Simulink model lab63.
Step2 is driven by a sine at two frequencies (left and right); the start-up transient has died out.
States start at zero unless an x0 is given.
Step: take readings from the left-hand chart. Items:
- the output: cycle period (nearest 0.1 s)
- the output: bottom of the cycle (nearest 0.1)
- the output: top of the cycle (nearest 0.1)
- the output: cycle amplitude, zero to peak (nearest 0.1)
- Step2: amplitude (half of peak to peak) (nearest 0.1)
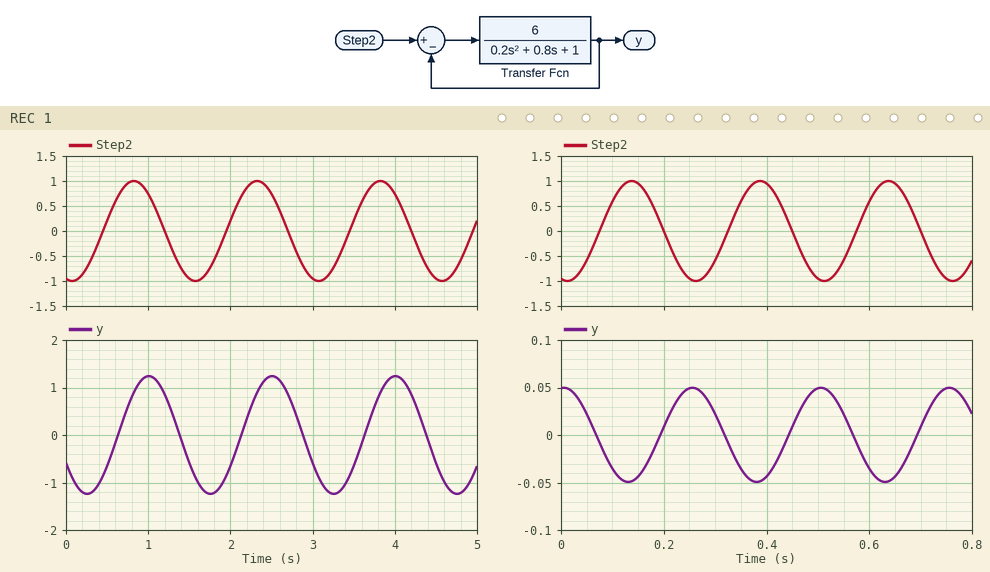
1.5 s
-1.2
1.2
1.2
1.0
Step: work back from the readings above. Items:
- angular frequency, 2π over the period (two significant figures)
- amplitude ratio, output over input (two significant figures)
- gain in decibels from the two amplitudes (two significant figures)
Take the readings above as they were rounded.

4.2 rad/s
1.2
1.6 dB
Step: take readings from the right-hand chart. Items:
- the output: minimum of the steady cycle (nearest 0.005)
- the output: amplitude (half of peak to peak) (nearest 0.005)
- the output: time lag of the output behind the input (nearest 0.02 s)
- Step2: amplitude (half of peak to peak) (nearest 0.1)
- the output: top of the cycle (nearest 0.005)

-0.050
0.050
0.12 s
1.0
0.050
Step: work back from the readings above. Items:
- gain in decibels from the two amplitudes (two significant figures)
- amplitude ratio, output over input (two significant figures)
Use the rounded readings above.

-26 dB
0.050
